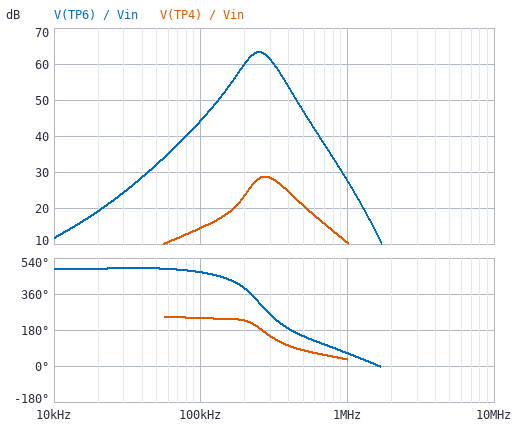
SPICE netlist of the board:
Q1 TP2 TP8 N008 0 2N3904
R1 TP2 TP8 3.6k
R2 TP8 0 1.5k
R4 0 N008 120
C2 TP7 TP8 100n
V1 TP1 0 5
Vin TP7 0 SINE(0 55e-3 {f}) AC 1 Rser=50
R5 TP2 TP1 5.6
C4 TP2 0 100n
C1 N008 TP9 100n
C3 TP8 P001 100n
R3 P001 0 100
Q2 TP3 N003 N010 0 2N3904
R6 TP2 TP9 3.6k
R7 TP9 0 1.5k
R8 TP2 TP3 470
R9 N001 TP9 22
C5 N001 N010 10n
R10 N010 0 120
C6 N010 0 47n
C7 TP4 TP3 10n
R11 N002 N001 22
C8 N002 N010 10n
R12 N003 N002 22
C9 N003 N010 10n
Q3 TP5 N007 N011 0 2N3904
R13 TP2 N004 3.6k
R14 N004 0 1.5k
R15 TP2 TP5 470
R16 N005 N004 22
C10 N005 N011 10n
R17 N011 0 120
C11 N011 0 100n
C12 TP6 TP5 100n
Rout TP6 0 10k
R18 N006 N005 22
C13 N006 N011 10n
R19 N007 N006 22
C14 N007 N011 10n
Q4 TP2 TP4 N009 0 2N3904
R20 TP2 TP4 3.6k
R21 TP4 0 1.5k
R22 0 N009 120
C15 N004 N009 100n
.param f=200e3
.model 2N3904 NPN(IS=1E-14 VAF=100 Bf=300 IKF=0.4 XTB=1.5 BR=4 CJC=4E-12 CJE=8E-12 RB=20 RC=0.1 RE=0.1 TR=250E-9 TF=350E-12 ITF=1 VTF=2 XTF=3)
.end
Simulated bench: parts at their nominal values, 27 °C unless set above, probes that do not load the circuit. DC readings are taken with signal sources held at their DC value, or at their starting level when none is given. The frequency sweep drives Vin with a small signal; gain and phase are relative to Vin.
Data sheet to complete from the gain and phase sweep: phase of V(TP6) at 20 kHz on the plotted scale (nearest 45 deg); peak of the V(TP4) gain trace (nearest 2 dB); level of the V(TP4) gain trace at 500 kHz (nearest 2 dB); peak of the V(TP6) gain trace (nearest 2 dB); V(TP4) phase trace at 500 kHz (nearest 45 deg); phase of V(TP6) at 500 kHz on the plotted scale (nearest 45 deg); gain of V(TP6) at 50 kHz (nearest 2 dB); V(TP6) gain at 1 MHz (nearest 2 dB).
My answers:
495 deg
28 dB
20 dB
64 dB
90 deg
135 deg
32 dB
28 dB
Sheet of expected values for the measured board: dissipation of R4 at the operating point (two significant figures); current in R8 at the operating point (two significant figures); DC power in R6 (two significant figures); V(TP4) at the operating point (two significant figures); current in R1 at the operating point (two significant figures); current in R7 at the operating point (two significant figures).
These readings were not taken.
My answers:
4.1 mW
5.8 mA
3.3 mW
1.4 V
960 µA
940 µA
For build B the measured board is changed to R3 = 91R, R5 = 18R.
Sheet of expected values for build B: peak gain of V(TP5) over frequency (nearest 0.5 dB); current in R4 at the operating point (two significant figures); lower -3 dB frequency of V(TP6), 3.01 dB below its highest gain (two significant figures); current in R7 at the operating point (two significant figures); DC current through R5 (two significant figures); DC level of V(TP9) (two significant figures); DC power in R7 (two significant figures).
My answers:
61.0 dB
5.2 mA
190 kHz
880 µA
24 mA
1.3 V
1.2 mW
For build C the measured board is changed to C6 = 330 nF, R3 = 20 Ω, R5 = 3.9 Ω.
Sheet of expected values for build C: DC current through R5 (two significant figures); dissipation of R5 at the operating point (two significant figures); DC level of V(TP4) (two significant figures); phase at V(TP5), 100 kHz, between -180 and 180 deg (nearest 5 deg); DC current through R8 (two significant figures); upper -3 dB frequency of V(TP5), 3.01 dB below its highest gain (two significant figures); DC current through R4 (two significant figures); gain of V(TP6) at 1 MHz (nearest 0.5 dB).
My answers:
28 mA
3.0 mW
1.4 V
35 deg
5.9 mA
250 kHz
6.0 mA
21.0 dB
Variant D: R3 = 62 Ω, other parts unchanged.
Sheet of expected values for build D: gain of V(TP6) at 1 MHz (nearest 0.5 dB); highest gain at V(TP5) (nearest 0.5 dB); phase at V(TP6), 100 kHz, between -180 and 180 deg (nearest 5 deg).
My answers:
26.0 dB
61.5 dB
105 deg
